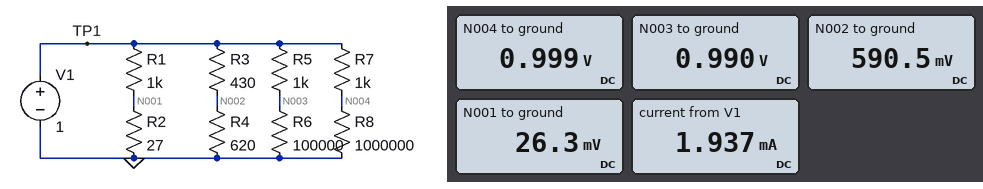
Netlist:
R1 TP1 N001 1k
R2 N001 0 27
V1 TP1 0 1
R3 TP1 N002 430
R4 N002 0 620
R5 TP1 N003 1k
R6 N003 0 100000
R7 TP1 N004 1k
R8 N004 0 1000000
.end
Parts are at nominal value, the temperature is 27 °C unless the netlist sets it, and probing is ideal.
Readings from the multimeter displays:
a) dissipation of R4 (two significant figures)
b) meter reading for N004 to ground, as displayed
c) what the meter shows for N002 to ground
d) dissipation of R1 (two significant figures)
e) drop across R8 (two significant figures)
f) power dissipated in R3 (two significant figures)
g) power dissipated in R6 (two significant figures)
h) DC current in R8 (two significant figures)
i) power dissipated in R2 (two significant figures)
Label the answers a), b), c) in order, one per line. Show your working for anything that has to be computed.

a) (590.5 mV)^2 / 620 Ω = 560 µW
b) 0.999 V
c) 590.5 mV
d) (1 V - 26.3 mV)^2 / 1 kΩ = 950 µW
e) 999 mV = 1.0 V
f) (1 V - 590.5 mV)^2 / 430 Ω = 390 µW
g) (990 mV)^2 / 100 kΩ = 9.8 µW
h) (999 mV) / 1 MΩ = 1.0 µA
i) (26.3 mV)^2 / 27 Ω = 26 µW
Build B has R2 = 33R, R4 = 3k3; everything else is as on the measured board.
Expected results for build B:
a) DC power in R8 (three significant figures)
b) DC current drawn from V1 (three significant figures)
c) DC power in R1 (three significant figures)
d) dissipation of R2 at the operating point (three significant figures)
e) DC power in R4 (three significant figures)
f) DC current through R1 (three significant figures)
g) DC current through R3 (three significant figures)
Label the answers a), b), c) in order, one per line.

a) 998 nW
b) 1.25 mA
c) 937 µW
d) 30.9 µW
e) 237 µW
f) 968 µA
g) 268 µA
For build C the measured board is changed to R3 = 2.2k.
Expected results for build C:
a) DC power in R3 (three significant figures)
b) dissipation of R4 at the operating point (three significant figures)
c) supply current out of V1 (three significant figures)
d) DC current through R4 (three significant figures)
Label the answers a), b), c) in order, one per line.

a) 277 µW
b) 78.0 µW
c) 1.34 mA
d) 355 µA
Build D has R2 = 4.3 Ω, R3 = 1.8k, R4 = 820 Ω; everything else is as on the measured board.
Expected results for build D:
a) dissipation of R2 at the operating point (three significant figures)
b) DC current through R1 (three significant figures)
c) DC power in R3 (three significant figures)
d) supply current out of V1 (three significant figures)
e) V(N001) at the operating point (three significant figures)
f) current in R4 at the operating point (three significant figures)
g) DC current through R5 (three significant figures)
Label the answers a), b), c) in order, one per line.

a) 4.26 µW
b) 996 µA
c) 262 µW
d) 1.39 mA
e) 4.28 mV
f) 382 µA
g) 9.90 µA
